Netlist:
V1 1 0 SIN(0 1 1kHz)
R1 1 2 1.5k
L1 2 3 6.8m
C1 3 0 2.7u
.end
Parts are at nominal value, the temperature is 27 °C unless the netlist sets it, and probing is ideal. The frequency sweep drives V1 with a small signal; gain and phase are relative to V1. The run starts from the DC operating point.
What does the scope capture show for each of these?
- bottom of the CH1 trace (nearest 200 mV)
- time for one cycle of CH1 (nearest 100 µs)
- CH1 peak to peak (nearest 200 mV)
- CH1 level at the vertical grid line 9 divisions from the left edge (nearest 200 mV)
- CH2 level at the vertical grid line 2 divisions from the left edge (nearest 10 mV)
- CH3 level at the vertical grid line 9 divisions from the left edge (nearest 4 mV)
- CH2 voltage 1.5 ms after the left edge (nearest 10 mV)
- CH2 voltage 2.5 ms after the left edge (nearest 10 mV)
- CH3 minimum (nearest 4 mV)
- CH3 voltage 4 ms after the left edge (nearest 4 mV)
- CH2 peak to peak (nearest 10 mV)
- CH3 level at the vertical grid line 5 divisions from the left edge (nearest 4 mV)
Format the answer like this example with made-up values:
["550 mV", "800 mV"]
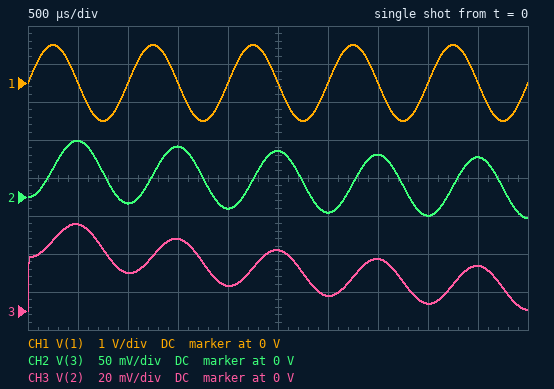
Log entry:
["-1.0 V", "1.0 ms", "2.0 V", "0 V", "-10 mV", "24 mV", "70 mV", "60 mV", "0 V", "4 mV", "100 mV", "32 mV"]
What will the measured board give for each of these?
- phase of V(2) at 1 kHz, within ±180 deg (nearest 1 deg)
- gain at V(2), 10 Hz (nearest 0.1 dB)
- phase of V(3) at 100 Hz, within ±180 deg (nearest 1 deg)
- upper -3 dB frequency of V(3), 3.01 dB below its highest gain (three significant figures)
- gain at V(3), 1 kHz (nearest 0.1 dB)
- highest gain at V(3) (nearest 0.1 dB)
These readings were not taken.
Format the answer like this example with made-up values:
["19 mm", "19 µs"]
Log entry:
["-89 deg", "-0.3 dB", "-69 deg", "39.3 Hz", "-28.1 dB", "0 dB"]
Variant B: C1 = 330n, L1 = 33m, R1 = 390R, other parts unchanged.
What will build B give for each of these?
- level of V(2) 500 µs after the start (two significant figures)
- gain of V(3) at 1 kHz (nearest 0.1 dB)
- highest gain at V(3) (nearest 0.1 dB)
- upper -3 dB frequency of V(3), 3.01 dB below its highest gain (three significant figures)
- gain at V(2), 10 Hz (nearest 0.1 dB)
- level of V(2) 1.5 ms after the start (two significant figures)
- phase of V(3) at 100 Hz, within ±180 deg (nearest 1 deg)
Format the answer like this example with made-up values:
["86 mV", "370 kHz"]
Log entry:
["420 mV", "0.1 dB", "0.3 dB", "1.68 kHz", "0 dB", "470 mV", "-5 deg"]
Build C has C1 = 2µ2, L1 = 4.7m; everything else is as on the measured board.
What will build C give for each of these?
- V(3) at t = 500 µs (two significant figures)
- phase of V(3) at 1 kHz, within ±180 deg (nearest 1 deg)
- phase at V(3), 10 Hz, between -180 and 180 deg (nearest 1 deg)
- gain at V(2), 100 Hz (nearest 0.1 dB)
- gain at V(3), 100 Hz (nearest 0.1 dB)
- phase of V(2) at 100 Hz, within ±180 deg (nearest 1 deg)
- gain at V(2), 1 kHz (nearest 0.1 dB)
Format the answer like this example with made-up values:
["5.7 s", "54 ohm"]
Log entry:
["90 mV", "-88 deg", "-12 deg", "-7.3 dB", "-7.2 dB", "-64 deg", "-30.9 dB"]
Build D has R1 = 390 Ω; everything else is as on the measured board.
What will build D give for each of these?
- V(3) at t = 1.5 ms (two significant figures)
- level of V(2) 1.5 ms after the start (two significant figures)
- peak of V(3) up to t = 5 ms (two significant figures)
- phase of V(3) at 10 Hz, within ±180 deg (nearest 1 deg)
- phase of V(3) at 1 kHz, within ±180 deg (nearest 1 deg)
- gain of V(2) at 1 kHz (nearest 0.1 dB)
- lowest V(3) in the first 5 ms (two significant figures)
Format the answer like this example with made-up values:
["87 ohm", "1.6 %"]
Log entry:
["190 mV", "78 mV", "250 mV", "-4 deg", "-88 deg", "-27.6 dB", "-150 mV"]
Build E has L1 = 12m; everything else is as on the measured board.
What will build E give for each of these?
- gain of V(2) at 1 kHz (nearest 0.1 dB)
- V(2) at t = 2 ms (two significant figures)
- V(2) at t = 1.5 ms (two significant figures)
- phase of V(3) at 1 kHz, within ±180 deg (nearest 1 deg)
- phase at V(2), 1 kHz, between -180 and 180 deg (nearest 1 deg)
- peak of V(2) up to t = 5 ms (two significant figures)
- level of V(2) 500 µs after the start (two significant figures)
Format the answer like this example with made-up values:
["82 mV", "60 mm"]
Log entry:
["-39.2 dB", "35 mV", "16 mV", "-91 deg", "89 deg", "49 mV", "24 mV"]
